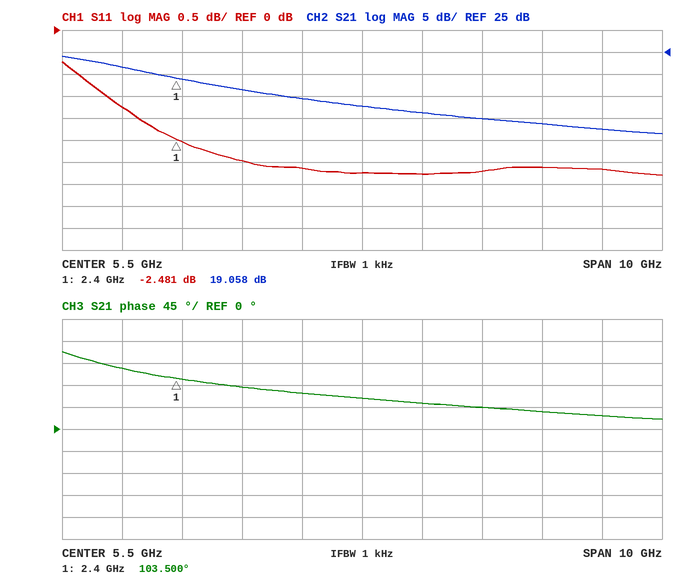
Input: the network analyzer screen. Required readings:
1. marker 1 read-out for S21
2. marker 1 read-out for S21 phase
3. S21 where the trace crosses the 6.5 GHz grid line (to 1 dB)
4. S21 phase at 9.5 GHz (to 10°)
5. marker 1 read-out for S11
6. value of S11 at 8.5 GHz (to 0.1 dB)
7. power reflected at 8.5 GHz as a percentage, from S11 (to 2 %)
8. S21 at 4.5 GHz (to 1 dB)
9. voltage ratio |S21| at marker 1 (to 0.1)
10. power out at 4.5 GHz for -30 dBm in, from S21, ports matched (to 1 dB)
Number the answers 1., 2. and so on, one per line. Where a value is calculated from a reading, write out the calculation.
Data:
1. 19.058 dB
2. 103.500°
3. 11 dB
4. 30°
5. -2.481 dB
6. -3.1 dB
7. 10^(-3.1/10) ≈ 49.0 %, so 48 % to the nearest 2 %
8. 14 dB
9. 10^(19.058/20) ≈ 9.0
10. -30 dBm + (14 dB) = -16 dBm
